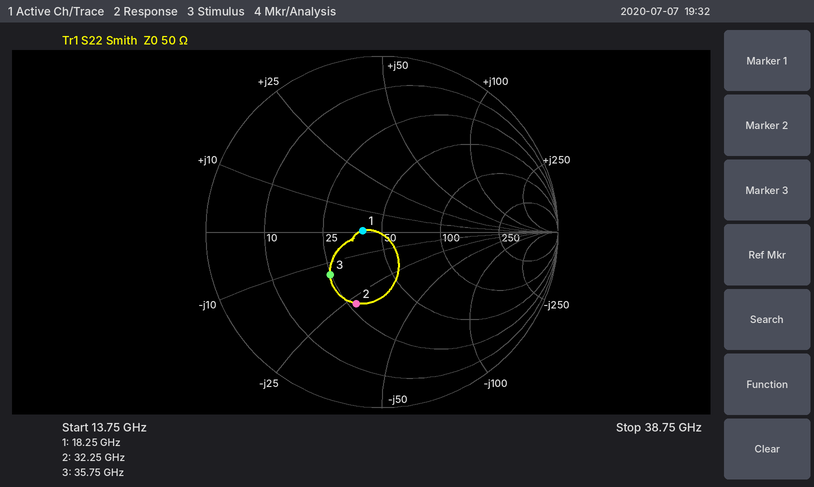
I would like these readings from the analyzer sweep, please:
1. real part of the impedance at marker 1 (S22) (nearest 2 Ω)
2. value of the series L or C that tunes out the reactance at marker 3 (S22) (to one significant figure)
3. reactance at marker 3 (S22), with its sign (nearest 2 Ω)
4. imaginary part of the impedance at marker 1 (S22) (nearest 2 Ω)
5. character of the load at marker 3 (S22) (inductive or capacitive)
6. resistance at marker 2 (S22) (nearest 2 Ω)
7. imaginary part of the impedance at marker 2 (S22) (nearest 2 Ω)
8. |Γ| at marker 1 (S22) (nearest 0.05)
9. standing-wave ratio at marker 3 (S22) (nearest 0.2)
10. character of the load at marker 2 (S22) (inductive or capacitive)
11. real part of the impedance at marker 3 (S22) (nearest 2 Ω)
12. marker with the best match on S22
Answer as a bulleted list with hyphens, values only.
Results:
- 40 Ω
- 60 pH
- -14 Ω
- 0 Ω
- capacitive
- 28 Ω
- -28 Ω
- 0.10
- 2.2
- capacitive
- 24 Ω
- marker 1
